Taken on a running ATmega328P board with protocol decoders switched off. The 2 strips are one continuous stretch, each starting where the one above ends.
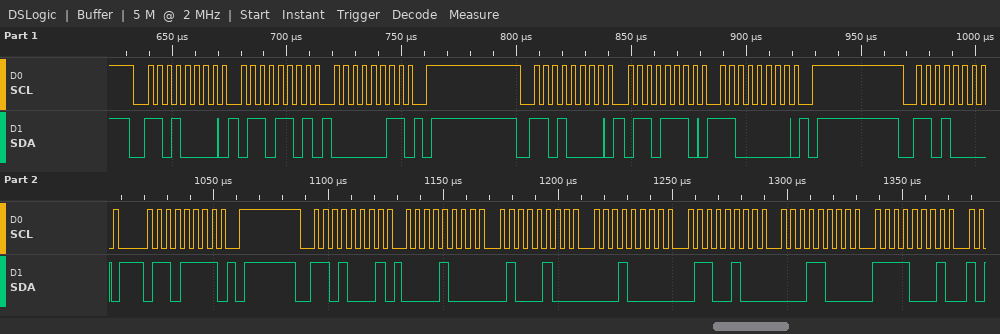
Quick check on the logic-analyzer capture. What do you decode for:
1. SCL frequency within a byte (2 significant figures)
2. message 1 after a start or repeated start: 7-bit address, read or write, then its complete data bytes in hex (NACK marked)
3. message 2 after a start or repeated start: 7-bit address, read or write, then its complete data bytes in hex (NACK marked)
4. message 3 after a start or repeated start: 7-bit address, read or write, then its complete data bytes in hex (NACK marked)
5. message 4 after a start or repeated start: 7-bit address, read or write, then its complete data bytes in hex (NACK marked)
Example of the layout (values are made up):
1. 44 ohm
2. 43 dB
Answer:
1. 250 kHz
2. 0x68 write: 6D 03
3. 0x68 write: 6E C0
4. 0x68 write: 6F
5. 0x68 read: 08 44 10 64 18 F1
